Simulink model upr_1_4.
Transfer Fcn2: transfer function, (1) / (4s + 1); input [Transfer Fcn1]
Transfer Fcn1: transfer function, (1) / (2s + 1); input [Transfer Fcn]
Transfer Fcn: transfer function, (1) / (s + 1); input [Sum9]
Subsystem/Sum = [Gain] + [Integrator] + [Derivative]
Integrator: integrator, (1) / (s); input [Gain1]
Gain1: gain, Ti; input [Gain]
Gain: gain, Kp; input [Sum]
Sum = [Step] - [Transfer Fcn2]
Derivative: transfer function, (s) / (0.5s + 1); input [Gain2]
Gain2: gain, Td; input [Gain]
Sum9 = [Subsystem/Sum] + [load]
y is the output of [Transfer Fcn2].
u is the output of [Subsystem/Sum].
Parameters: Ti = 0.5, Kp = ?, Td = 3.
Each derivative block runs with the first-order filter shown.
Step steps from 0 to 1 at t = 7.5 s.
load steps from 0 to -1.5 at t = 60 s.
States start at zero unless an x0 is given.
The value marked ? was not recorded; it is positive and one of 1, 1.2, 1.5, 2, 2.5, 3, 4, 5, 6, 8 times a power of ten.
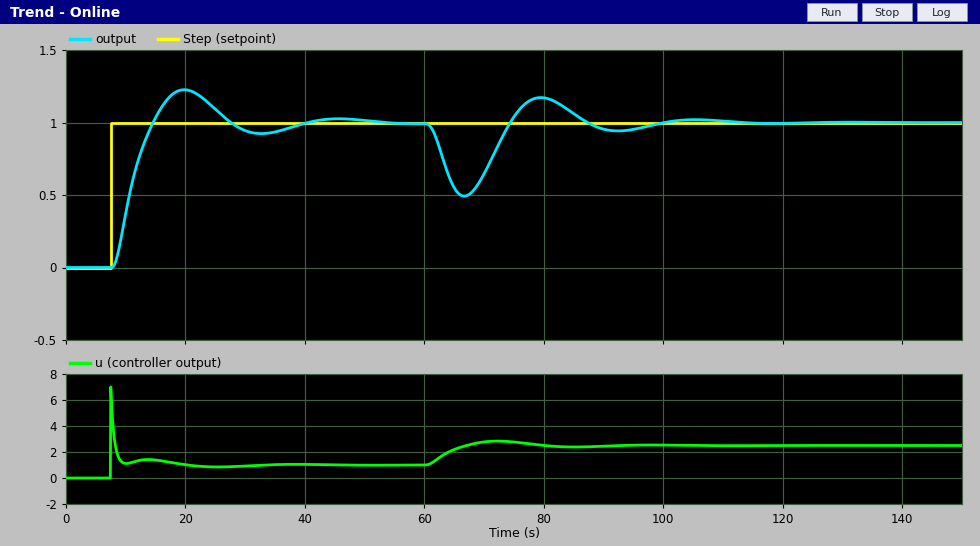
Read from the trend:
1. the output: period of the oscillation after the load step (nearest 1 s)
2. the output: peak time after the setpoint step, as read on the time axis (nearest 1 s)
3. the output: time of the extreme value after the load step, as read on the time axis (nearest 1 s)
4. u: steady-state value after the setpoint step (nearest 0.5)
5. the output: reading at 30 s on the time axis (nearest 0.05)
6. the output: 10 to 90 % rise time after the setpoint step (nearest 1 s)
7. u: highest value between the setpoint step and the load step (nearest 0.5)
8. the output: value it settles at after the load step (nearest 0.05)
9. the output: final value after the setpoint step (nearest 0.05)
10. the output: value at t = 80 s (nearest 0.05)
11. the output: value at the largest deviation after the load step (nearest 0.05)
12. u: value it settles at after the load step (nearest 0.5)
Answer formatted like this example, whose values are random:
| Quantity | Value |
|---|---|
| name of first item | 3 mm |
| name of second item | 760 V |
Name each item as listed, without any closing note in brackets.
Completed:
| Quantity | Value |
|---|---|
| the output: period of the oscillation after the load step | 26 s |
| the output: peak time after the setpoint step, as read on the time axis | 20 s |
| the output: time of the extreme value after the load step, as read on the time axis | 67 s |
| u: steady-state value after the setpoint step | 1.0 |
| the output: reading at 30 s on the time axis | 0.95 |
| the output: 10 to 90 % rise time after the setpoint step | 5 s |
| u: highest value between the setpoint step and the load step | 7.0 |
| the output: value it settles at after the load step | 1.00 |
| the output: final value after the setpoint step | 1.00 |
| the output: value at t = 80 s | 1.15 |
| the output: value at the largest deviation after the load step | 0.50 |
| u: value it settles at after the load step | 2.5 |
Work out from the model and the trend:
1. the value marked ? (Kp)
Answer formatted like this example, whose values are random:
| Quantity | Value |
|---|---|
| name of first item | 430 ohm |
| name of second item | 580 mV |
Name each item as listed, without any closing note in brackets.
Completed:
| Quantity | Value |
|---|---|
| the value marked ? | 1 |
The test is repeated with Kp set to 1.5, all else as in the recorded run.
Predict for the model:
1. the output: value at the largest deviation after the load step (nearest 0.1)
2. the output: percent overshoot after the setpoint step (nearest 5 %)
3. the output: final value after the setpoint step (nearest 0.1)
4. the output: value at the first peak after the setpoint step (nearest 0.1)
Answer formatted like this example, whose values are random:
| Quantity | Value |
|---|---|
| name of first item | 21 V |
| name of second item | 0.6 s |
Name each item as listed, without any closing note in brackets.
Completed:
| Quantity | Value |
|---|---|
| the output: value at the largest deviation after the load step | 0.6 |
| the output: percent overshoot after the setpoint step | 20 % |
| the output: final value after the setpoint step | 1.0 |
| the output: value at the first peak after the setpoint step | 1.2 |
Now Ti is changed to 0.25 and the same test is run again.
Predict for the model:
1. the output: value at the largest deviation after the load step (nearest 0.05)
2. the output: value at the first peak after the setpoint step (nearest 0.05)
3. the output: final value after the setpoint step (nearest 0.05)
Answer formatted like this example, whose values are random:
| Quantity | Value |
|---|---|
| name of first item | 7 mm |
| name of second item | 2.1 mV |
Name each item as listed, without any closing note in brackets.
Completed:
| Quantity | Value |
|---|---|
| the output: value at the largest deviation after the load step | 0.45 |
| the output: value at the first peak after the setpoint step | 1.05 |
| the output: final value after the setpoint step | 1.00 |
